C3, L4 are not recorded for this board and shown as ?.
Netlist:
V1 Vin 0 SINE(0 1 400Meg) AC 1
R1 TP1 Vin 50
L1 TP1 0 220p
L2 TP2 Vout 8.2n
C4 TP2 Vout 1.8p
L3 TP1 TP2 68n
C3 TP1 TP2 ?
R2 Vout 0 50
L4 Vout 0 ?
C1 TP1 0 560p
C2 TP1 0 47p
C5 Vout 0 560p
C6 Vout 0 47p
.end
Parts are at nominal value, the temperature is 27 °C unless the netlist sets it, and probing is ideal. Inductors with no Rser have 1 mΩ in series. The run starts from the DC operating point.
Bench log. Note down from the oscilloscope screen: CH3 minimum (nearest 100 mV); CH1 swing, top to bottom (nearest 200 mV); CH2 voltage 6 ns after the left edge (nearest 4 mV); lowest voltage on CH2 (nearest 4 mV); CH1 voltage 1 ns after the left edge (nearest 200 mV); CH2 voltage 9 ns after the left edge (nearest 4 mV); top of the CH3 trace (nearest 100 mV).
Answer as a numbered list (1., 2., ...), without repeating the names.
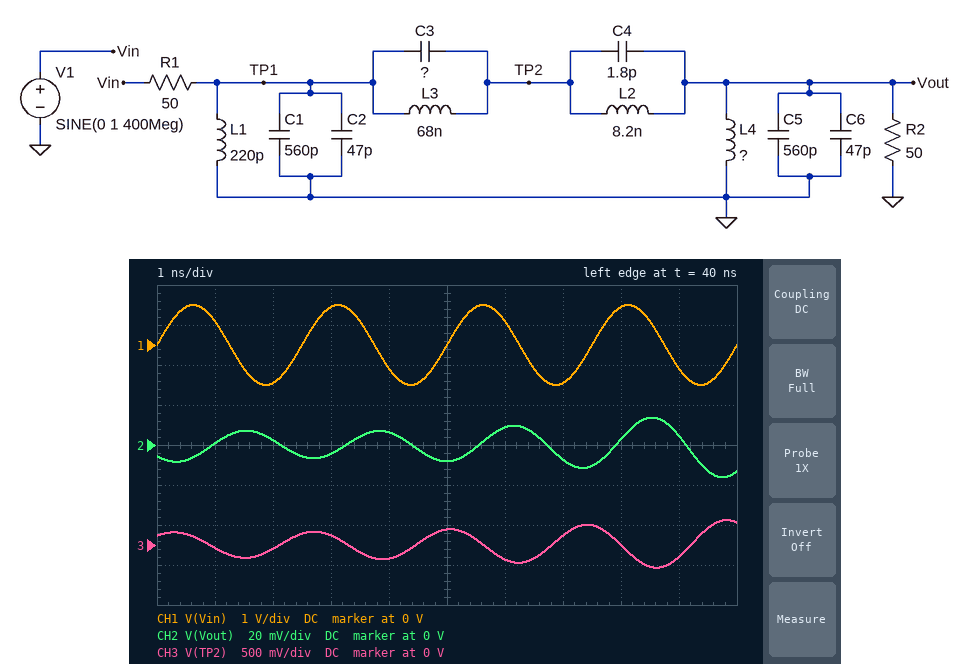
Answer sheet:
1. -300 mV
2. 2.0 V
3. 8 mV
4. -16 mV
5. 600 mV
6. 4 mV
7. 300 mV
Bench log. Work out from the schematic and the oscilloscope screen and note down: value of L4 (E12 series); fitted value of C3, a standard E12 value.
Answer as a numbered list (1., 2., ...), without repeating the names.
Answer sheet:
1. 560 pH
2. 22 pF
